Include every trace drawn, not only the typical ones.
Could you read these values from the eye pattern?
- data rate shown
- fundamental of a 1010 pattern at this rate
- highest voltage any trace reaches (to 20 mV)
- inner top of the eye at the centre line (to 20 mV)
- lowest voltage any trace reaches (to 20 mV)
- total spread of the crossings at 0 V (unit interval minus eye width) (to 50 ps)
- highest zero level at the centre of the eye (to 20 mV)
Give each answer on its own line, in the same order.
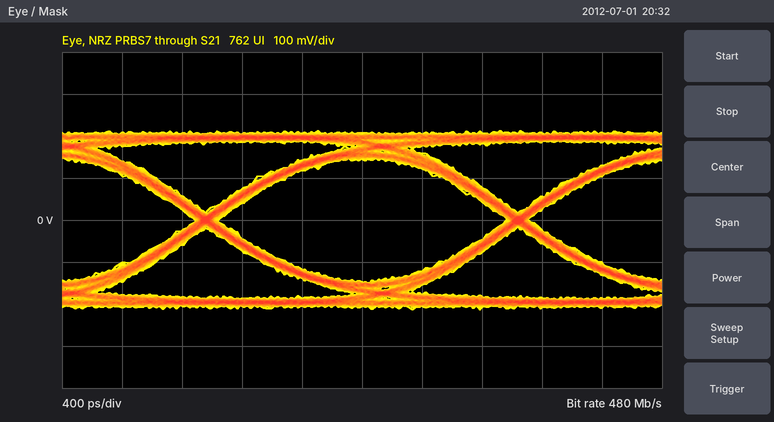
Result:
480 Mb/s
240 MHz
220 mV
140 mV
-220 mV
150 ps
-140 mV
